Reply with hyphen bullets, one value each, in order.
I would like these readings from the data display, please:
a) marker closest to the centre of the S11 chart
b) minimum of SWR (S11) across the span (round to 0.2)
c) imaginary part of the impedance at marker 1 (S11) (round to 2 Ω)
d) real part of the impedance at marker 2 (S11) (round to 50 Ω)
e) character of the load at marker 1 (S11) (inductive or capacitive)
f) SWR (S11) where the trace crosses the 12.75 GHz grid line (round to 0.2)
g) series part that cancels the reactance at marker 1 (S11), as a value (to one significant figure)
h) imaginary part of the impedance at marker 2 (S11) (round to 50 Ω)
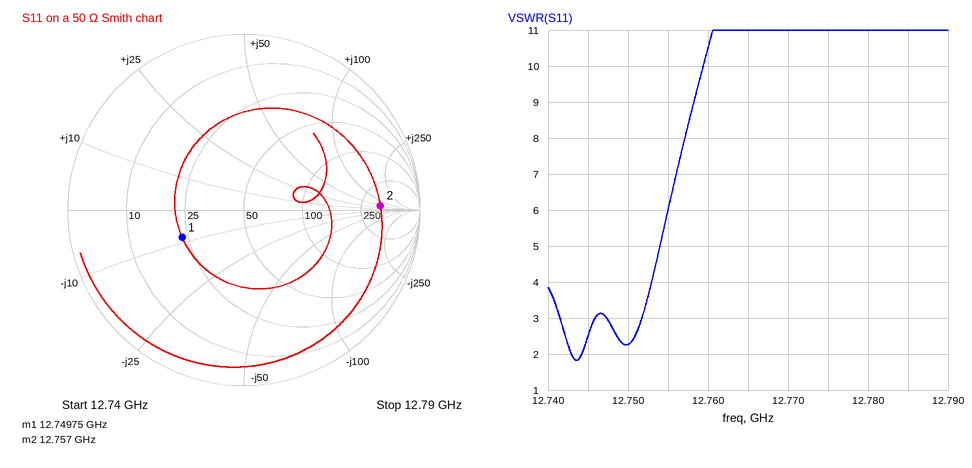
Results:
- marker 1
- 1.8
- -8 Ω
- 400 Ω
- capacitive
- 2.2
- 100 pH
- +50 Ω
